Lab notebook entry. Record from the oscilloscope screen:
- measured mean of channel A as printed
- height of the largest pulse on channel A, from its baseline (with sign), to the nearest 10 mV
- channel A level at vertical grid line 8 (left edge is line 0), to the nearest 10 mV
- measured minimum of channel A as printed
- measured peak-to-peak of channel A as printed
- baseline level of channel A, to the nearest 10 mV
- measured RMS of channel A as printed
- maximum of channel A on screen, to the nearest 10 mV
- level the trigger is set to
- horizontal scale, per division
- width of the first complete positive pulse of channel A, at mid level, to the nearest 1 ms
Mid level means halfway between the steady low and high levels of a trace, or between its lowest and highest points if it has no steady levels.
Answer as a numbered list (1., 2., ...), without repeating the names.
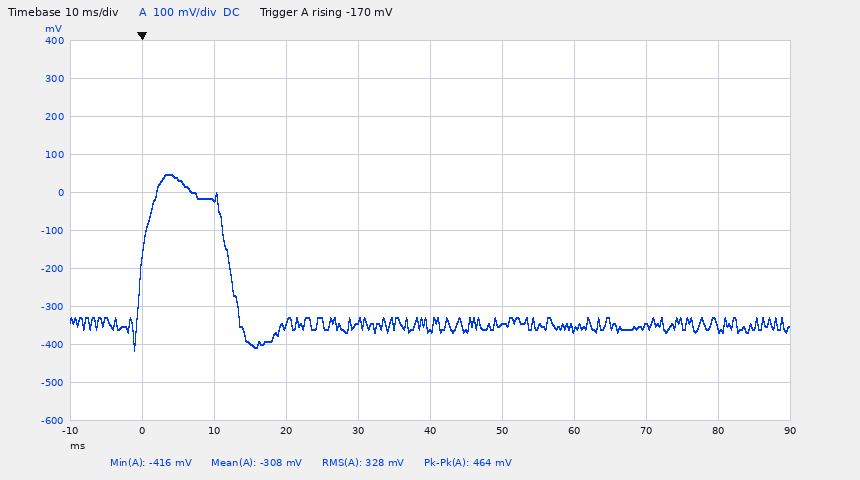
1. -308 mV
2. +400 mV
3. -350 mV
4. -416 mV
5. 464 mV
6. -350 mV
7. 328 mV
8. 50 mV
9. -170 mV
10. 10 ms
11. 12 ms
